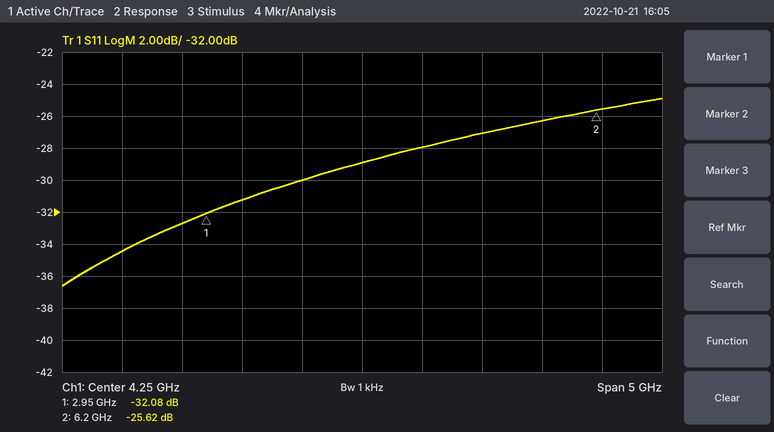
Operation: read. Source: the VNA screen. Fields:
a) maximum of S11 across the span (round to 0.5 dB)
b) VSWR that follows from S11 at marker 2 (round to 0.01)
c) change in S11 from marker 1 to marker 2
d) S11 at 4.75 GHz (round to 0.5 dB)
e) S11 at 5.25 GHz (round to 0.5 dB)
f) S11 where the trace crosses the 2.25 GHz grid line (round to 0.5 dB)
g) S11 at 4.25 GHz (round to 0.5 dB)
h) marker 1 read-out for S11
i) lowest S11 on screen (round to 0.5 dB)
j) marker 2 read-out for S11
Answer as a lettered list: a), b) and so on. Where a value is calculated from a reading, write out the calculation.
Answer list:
a) -25.0 dB
b) (1 + 0.0524)/(1 − 0.0524) ≈ 1.11
c) -25.62 − (-32.08) = 6.46 dB
d) -28.0 dB
e) -27.0 dB
f) -34.5 dB
g) -29.0 dB
h) -32.08 dB
i) -36.5 dB
j) -25.62 dB
